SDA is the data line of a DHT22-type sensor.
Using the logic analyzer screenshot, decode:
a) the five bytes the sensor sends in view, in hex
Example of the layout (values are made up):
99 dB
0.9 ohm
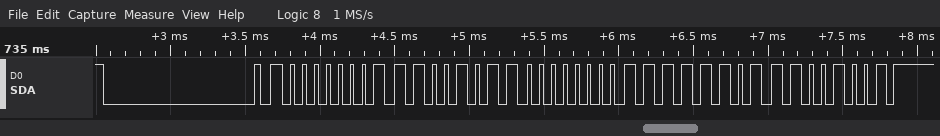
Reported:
01, CB, 00, FD, C9
